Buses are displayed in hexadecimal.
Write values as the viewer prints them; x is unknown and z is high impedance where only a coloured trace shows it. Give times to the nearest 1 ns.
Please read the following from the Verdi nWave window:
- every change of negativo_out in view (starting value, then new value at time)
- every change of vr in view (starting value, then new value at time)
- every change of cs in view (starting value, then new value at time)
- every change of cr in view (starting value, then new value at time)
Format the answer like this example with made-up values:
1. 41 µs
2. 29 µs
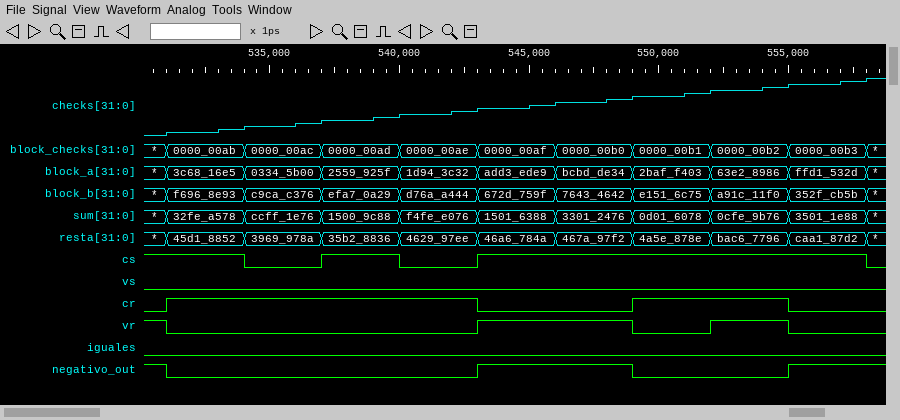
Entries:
1. 1, 0 at 531 ns, 1 at 543 ns, 0 at 549 ns, 1 at 555 ns
2. 1, 0 at 531 ns, 1 at 543 ns, 0 at 549 ns, 1 at 552 ns, 0 at 555 ns
3. 1, 0 at 534 ns, 1 at 537 ns, 0 at 540 ns, 1 at 543 ns, 0 at 558 ns
4. 0, 1 at 531 ns, 0 at 543 ns, 1 at 549 ns, 0 at 555 ns
